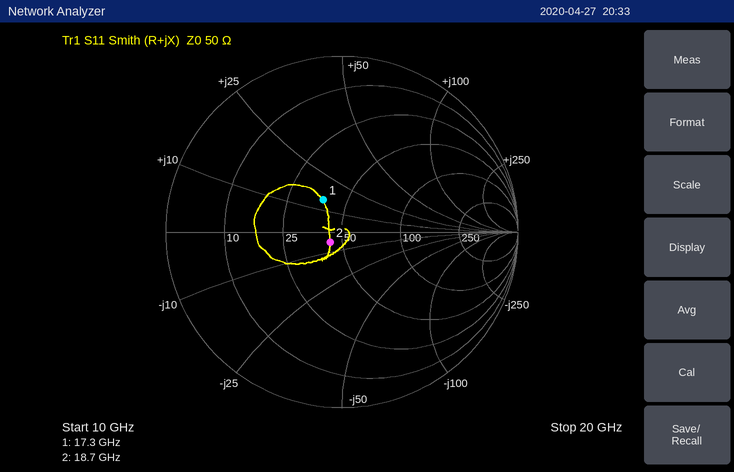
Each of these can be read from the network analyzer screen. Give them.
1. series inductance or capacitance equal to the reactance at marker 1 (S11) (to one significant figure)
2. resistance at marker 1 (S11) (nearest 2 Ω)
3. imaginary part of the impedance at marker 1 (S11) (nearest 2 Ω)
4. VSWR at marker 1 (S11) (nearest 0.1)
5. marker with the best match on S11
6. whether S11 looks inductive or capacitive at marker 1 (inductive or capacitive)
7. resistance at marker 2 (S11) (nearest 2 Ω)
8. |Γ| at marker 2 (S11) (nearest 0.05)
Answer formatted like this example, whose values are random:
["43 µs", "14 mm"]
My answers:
["100 pH", "38 Ω", "+14 Ω", "1.5", "marker 2", "inductive", "44 Ω", "0.10"]
